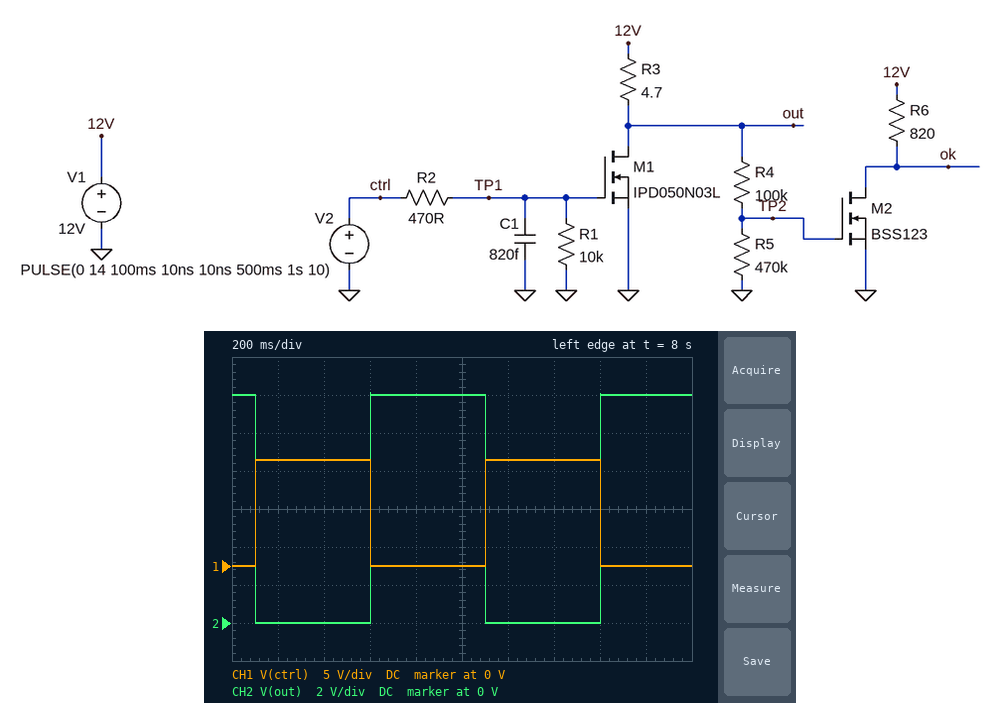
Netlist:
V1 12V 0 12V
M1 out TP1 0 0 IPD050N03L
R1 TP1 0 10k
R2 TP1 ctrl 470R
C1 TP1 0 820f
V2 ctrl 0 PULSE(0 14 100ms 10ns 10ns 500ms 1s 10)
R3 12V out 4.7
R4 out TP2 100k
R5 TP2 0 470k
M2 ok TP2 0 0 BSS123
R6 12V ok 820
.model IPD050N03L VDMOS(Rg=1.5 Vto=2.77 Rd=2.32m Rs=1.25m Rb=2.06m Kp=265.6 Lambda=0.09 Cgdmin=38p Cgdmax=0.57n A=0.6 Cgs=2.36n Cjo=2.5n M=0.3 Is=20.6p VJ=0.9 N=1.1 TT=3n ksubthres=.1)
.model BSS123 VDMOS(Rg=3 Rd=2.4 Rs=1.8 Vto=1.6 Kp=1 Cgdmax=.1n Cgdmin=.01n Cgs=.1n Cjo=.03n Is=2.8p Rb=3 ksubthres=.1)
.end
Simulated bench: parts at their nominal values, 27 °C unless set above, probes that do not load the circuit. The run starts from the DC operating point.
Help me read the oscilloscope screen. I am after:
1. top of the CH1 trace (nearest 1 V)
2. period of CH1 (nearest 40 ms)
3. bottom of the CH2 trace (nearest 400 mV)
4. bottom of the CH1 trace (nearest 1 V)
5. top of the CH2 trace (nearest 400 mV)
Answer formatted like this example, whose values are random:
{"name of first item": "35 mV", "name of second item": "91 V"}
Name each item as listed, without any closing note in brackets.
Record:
{"top of the CH1 trace": "14 V", "period of CH1": "1.00 s", "bottom of the CH2 trace": "0 V", "bottom of the CH1 trace": "0 V", "top of the CH2 trace": "12.0 V"}
